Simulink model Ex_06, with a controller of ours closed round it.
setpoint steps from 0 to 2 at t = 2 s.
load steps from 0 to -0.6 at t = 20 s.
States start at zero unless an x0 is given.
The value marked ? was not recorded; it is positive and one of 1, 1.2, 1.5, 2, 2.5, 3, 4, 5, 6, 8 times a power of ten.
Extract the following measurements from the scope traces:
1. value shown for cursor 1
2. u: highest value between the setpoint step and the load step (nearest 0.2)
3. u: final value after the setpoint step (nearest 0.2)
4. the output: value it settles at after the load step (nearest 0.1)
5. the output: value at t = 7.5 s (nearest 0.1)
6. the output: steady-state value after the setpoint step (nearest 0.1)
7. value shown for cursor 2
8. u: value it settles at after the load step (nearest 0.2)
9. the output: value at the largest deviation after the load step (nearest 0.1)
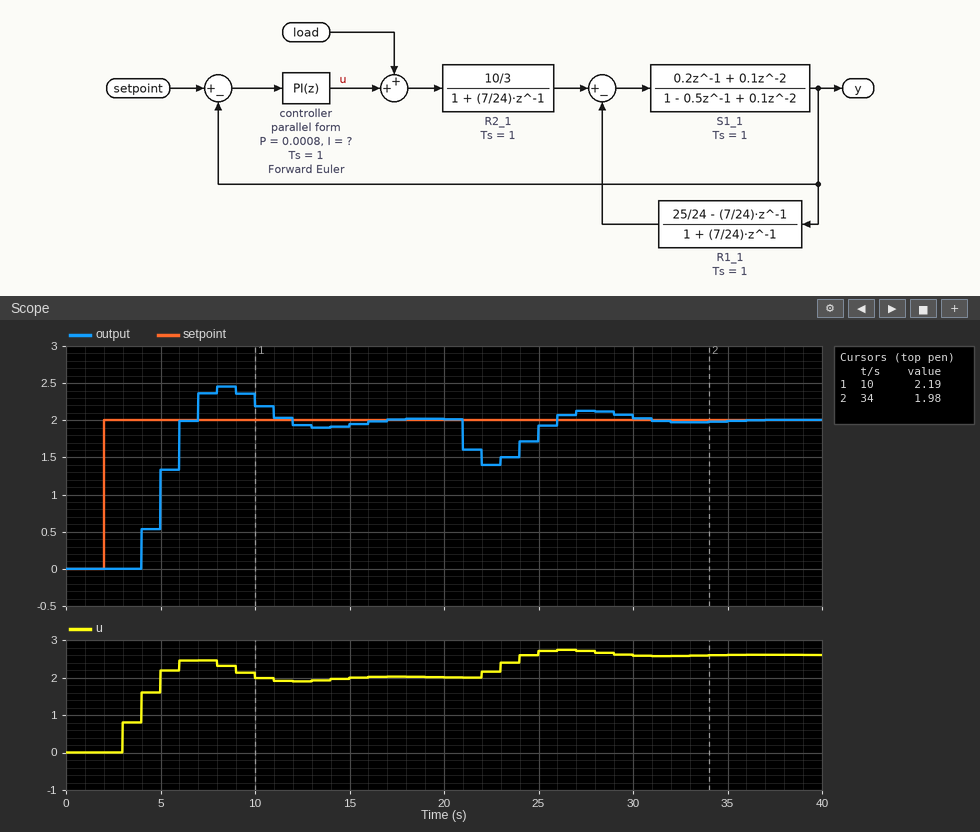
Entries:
2.19
2.4
2.0
2.0
2.4
2.0
1.98
2.6
1.4
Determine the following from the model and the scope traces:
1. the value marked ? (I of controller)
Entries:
0.4
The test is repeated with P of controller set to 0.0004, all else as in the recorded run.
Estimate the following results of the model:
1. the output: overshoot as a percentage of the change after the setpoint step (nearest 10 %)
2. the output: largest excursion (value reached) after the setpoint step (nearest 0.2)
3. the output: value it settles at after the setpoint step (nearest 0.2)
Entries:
20 %
2.4
2.0
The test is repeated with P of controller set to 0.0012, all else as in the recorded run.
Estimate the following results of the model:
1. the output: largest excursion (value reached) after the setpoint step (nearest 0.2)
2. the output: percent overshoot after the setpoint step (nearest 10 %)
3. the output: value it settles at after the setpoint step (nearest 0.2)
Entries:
2.4
20 %
2.0
